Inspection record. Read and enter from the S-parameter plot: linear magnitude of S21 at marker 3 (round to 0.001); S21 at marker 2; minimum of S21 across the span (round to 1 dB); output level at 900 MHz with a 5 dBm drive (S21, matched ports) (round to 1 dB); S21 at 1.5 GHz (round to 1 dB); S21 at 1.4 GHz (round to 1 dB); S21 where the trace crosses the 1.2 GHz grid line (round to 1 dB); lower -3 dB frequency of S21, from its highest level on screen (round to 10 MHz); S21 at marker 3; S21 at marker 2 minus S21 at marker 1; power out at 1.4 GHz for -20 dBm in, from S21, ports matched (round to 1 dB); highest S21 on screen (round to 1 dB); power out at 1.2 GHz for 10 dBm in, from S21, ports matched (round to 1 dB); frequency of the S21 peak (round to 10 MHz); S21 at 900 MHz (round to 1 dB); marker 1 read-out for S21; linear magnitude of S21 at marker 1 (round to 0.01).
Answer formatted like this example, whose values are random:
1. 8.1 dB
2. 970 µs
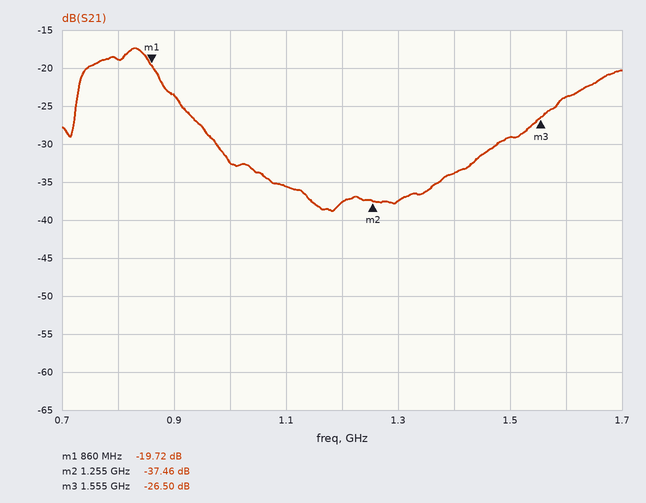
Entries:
1. 0.047
2. -37.46 dB
3. -39 dB
4. -19 dBm
5. -29 dB
6. -34 dB
7. -38 dB
8. 740 MHz
9. -26.50 dB
10. -17.74 dB
11. -54 dBm
12. -17 dB
13. -28 dBm
14. 830 MHz
15. -24 dB
16. -19.72 dB
17. 0.10
